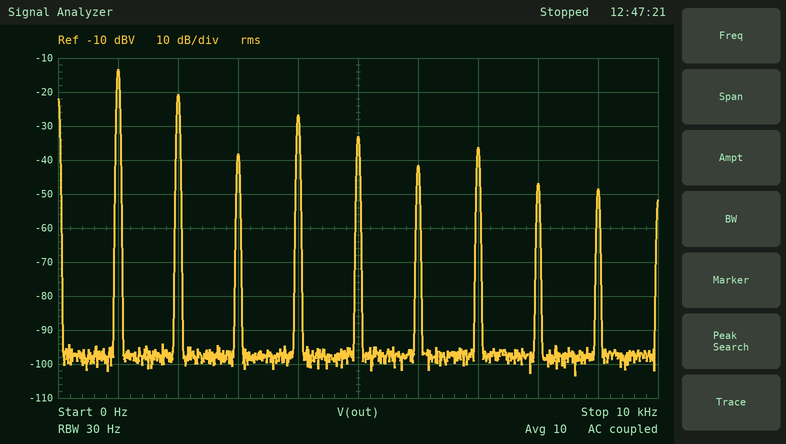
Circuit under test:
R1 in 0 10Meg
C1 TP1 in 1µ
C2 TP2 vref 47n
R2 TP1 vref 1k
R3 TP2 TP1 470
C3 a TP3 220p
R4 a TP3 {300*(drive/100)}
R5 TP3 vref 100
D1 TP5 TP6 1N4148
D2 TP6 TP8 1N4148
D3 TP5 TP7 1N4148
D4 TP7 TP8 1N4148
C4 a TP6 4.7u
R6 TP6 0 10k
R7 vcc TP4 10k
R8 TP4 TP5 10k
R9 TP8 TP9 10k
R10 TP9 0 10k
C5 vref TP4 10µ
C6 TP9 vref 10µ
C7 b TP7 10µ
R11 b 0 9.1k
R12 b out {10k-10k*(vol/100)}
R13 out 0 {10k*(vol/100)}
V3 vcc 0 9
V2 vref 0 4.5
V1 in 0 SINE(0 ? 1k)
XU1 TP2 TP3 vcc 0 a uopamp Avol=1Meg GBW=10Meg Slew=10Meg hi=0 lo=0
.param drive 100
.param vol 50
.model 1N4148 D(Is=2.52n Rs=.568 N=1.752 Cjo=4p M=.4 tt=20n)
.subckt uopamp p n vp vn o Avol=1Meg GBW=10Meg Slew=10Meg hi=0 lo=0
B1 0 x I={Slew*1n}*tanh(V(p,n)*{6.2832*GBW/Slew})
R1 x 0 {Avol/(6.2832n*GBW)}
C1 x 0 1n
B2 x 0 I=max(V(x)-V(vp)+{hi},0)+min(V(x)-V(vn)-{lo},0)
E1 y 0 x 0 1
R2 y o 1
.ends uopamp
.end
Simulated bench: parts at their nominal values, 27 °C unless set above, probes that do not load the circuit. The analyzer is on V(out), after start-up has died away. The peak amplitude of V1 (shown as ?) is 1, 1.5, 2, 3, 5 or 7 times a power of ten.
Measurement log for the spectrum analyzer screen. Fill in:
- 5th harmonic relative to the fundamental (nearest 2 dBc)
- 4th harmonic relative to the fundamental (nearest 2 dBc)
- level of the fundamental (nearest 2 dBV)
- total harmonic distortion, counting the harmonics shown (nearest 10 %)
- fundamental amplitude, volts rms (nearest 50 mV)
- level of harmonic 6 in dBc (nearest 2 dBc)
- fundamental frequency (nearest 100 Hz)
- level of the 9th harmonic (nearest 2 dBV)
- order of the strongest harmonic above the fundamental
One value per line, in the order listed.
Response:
-20 dBc
-14 dBc
-14 dBV
50 %
200 mV
-28 dBc
1.0 kHz
-48 dBV
2
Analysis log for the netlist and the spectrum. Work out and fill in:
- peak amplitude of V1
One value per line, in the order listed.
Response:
700 mV
